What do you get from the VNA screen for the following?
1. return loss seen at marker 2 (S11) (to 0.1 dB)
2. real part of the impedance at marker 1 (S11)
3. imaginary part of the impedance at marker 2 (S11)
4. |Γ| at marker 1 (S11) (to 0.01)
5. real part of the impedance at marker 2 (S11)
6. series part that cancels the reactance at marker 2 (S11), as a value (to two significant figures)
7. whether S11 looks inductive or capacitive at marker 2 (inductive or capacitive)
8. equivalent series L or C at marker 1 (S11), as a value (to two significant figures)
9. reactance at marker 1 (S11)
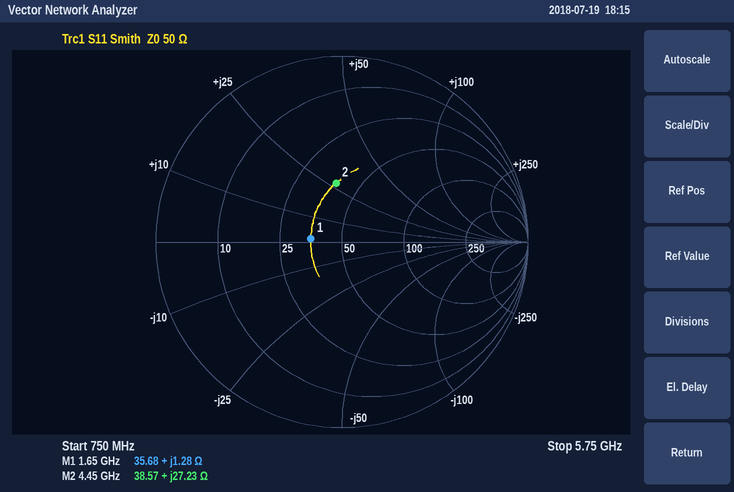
9.9 dB
35.68 Ω
+27.23 Ω
0.17
38.57 Ω
1.3 pF
inductive
120 pH
+1.28 Ω
